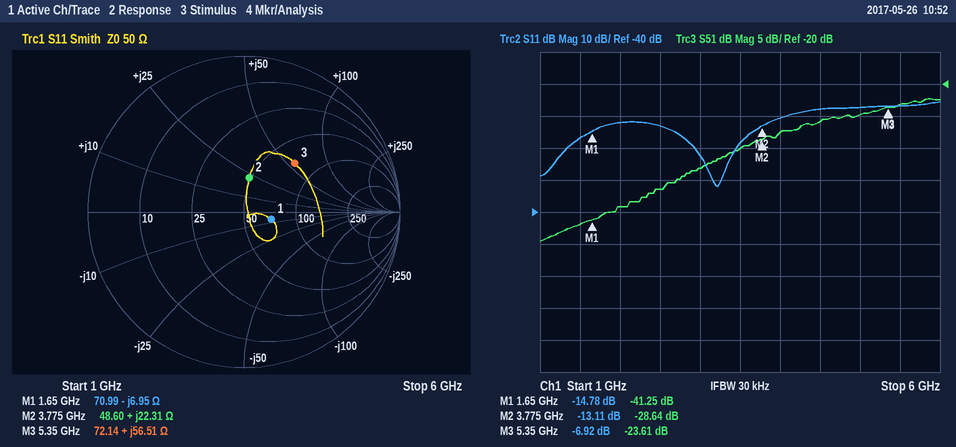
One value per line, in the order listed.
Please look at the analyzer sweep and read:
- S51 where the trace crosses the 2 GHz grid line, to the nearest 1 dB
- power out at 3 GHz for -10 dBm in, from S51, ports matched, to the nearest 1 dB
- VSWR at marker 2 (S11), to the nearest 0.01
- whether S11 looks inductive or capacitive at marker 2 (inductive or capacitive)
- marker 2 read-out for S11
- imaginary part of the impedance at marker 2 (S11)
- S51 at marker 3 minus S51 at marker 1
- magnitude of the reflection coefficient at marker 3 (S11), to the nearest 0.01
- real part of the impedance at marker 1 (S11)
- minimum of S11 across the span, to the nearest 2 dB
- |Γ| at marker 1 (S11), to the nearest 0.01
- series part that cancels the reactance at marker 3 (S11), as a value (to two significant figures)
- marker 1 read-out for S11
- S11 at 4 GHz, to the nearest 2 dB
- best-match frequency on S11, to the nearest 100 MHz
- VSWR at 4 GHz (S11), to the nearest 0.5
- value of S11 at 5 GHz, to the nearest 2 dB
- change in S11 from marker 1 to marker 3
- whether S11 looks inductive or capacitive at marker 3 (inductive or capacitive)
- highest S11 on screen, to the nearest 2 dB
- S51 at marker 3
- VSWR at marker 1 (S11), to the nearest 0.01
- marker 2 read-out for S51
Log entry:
-39 dB
-43 dBm
1.57
inductive
-13.11 dB
+22.31 Ω
17.64 dB
0.45
70.99 Ω
-32 dB
0.18
530 fF
-14.78 dB
-10 dB
3.2 GHz
2.0
-8 dB
7.86 dB
inductive
-6 dB
-23.61 dB
1.45
-28.64 dB
